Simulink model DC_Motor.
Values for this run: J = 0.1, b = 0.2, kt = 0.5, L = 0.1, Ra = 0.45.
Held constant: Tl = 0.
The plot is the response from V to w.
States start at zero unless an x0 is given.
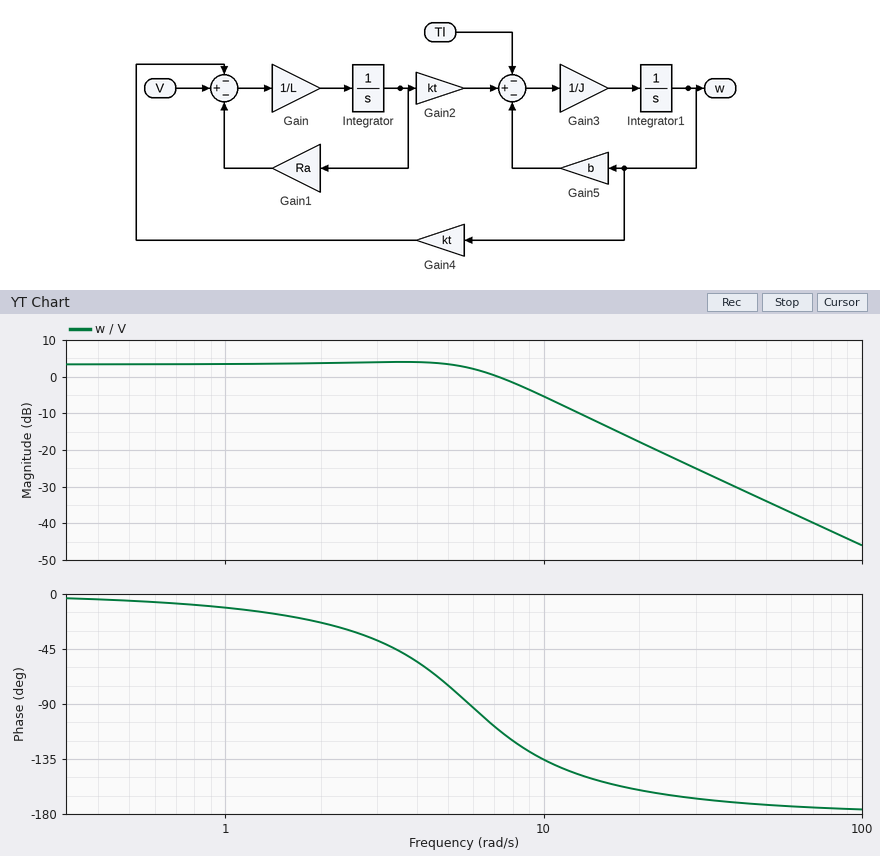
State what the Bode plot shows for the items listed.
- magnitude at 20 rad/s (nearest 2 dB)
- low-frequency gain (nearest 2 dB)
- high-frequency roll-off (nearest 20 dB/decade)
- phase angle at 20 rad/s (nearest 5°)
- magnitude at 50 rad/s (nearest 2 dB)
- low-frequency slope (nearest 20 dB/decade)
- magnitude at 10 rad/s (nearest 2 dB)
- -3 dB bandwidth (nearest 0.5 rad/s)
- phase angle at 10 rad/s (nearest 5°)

-18 dB
4 dB
-40 dB/decade
-160°
-34 dB
0 dB/decade
-6 dB
7.0 rad/s
-135°
